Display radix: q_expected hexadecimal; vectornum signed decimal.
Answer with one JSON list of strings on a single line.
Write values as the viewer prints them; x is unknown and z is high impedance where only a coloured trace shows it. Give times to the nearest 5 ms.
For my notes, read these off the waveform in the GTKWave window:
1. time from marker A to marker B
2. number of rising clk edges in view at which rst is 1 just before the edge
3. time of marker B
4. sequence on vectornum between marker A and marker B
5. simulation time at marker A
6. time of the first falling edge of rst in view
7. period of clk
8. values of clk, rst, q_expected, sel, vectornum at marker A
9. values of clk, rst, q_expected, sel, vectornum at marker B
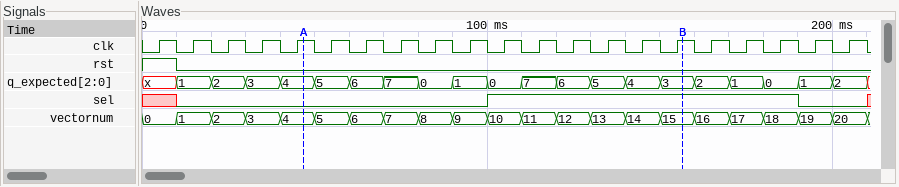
["110 ms", "1", "155 ms", "4, 5, 6, 7, 8, 9, 10, 11, 12, 13, 14, 15", "45 ms", "10 ms", "10 ms", "clk=1, rst=0, q_expected=4, sel=0, vectornum=4", "clk=1, rst=0, q_expected=3, sel=1, vectornum=15"]
